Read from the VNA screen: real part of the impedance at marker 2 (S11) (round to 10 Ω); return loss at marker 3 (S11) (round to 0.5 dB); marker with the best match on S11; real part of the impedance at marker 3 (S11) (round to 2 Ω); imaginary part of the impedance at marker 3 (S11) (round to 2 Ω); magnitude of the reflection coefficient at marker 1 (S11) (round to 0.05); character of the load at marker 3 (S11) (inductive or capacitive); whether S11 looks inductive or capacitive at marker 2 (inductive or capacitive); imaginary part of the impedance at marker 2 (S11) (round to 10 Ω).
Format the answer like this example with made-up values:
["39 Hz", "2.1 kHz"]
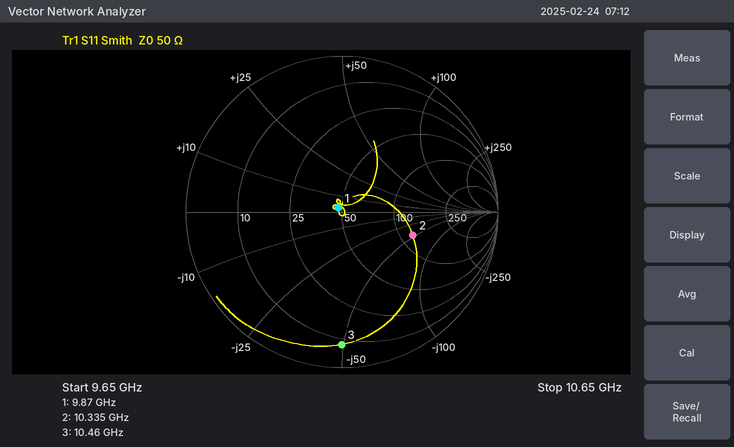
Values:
["120 Ω", "1.5 dB", "marker 1", "8 Ω", "-50 Ω", "0.05", "capacitive", "capacitive", "-50 Ω"]
